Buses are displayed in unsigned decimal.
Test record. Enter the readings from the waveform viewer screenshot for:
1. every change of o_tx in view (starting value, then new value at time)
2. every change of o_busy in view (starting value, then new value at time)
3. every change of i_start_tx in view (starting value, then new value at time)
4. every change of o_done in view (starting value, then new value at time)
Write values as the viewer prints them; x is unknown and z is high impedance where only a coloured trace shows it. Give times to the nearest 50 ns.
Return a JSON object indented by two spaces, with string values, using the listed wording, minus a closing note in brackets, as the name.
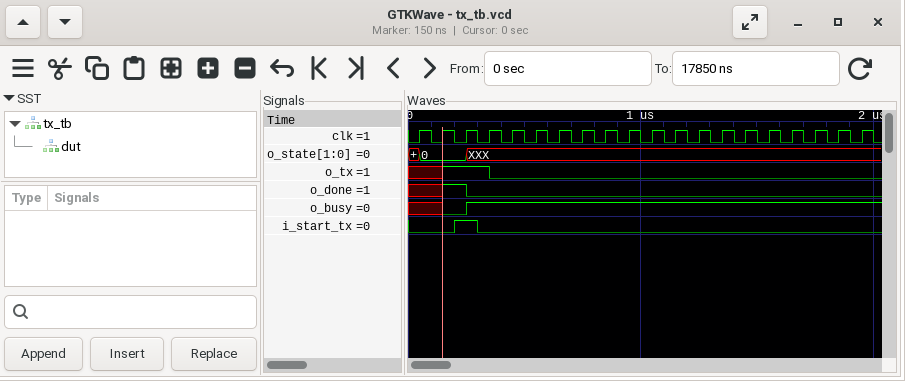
{
  "every change of o_tx in view": "x, 1 at 150 ns, 0 at 350 ns",
  "every change of o_busy in view": "x, 0 at 150 ns, 1 at 250 ns",
  "every change of i_start_tx in view": "0, 1 at 200 ns, 0 at 300 ns",
  "every change of o_done in view": "x, 1 at 150 ns, 0 at 250 ns"
}
